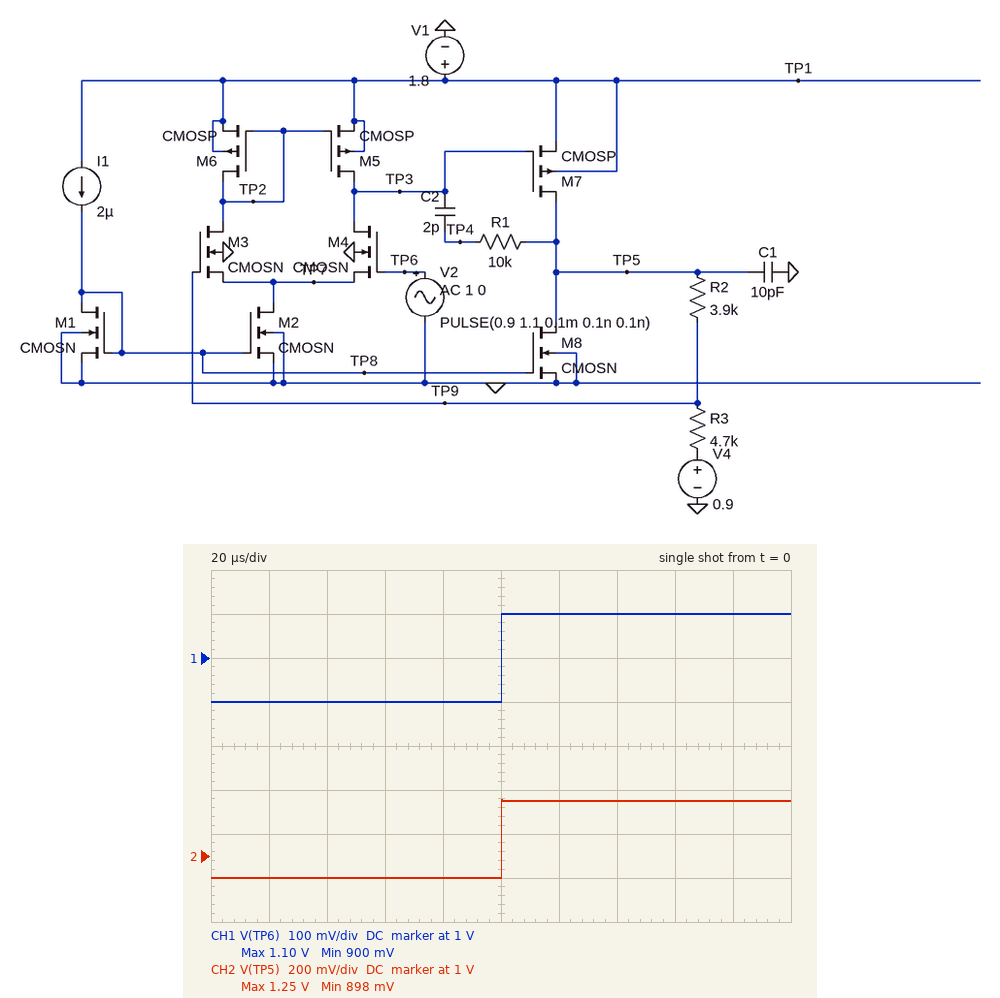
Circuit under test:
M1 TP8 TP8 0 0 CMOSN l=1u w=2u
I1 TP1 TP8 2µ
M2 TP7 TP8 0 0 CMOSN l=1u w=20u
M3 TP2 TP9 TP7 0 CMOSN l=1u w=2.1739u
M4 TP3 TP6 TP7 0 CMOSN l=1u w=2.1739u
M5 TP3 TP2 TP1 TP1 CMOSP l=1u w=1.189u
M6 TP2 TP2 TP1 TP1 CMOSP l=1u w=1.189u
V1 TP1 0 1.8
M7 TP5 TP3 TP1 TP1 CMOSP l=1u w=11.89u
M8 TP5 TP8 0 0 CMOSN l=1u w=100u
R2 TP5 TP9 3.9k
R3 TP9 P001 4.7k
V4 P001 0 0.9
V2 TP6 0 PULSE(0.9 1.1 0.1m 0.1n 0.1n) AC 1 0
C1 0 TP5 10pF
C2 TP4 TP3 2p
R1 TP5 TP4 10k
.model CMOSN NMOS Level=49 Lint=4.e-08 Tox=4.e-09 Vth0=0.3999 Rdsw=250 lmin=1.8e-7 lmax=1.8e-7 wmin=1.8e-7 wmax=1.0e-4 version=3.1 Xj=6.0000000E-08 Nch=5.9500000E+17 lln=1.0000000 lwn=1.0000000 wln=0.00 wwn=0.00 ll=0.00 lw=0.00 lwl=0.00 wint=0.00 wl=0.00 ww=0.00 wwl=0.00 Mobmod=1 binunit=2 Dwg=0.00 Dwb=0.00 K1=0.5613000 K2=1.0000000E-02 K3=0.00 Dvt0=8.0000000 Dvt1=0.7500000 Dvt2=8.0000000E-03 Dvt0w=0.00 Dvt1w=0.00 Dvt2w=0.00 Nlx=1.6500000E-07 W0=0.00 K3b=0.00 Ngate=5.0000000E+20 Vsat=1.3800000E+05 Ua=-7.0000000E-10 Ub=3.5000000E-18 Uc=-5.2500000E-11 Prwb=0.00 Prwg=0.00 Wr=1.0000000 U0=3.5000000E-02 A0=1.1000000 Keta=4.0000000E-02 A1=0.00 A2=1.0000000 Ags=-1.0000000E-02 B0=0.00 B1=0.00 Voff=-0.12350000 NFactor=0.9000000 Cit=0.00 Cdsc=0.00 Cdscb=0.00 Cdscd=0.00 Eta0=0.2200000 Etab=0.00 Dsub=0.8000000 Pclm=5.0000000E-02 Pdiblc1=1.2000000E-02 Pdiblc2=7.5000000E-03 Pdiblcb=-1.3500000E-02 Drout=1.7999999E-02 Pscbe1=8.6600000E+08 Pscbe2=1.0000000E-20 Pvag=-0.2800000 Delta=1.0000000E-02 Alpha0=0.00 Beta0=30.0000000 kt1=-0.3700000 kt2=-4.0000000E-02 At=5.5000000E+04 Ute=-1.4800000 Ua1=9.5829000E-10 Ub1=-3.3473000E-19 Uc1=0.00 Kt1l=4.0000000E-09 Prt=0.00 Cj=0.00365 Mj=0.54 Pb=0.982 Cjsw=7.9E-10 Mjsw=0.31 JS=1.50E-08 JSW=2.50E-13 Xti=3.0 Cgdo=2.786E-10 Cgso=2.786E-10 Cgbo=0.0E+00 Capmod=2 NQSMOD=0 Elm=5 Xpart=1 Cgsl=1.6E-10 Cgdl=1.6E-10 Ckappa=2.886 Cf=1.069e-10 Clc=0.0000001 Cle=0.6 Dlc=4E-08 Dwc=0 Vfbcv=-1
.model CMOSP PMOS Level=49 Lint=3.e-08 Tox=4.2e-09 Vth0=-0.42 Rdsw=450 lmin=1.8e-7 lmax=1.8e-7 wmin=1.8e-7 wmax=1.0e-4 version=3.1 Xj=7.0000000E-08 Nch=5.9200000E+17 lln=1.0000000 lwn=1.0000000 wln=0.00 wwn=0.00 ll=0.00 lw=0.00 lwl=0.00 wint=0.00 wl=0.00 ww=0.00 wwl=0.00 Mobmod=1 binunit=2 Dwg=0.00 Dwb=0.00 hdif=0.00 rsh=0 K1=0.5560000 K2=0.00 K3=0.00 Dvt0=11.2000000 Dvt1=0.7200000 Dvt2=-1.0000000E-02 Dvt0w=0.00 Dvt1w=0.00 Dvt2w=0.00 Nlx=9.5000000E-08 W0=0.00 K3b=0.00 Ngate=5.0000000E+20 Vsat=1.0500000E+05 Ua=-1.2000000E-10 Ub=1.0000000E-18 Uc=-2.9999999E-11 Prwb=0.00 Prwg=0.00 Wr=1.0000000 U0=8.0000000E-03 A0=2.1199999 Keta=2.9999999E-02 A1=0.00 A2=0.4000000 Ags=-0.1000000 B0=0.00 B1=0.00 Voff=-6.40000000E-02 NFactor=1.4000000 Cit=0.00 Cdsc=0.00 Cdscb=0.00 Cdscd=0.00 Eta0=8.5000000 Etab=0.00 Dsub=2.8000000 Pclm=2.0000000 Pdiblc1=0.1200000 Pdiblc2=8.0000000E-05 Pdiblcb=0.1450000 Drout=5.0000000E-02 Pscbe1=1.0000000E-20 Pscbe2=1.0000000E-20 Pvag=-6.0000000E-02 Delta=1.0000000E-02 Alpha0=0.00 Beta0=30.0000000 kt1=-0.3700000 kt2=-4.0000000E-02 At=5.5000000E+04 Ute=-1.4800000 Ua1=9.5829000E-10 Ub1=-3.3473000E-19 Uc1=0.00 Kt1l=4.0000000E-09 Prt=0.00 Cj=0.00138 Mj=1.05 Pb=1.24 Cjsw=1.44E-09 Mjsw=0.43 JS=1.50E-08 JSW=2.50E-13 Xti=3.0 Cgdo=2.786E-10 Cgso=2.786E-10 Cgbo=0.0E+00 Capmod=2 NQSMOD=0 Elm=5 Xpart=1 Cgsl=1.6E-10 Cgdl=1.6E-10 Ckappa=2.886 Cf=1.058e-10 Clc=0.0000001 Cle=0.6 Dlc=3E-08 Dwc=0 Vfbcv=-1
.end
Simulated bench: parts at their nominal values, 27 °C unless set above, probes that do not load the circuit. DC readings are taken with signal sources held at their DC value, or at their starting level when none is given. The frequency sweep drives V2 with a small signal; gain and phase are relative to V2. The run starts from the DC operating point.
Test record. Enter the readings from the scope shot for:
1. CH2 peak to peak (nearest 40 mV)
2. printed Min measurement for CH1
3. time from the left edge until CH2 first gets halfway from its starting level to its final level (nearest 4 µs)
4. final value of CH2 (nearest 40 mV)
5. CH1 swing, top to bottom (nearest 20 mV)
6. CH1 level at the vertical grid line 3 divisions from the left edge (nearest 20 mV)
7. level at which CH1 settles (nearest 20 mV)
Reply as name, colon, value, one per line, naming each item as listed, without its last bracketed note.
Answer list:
CH2 peak to peak: 360 mV
printed Min measurement for CH1: 900 mV
time from the left edge until CH2 first gets halfway from its starting level to its final level: 100 µs
final value of CH2: 1.24 V
CH1 swing, top to bottom: 200 mV
CH1 level at the vertical grid line 3 divisions from the left edge: 900 mV
level at which CH1 settles: 1.10 V
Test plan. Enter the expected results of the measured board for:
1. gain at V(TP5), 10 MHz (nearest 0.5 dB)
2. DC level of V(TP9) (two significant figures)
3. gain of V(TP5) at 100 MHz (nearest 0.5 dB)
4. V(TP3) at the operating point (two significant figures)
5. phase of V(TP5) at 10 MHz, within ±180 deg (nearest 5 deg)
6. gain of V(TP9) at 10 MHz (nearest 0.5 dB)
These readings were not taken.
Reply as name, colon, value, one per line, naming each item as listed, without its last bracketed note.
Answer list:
gain at V(TP5), 10 MHz: -10.5 dB
DC level of V(TP9): 900 mV
gain of V(TP5) at 100 MHz: -34.5 dB
V(TP3) at the operating point: 720 mV
phase of V(TP5) at 10 MHz, within ±180 deg: -100 deg
gain of V(TP9) at 10 MHz: -15.5 dB
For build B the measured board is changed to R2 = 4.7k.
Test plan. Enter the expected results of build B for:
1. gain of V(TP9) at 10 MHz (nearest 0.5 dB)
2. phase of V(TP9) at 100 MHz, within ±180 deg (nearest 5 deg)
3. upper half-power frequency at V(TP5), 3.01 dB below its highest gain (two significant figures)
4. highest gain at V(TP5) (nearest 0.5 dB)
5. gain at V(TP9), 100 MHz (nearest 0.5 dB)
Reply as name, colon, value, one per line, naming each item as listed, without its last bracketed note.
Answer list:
gain of V(TP9) at 10 MHz: -16.5 dB
phase of V(TP9) at 100 MHz, within ±180 deg: 150 deg
upper half-power frequency at V(TP5), 3.01 dB below its highest gain: 2.7 MHz
highest gain at V(TP5): 6.0 dB
gain at V(TP9), 100 MHz: -44.0 dB
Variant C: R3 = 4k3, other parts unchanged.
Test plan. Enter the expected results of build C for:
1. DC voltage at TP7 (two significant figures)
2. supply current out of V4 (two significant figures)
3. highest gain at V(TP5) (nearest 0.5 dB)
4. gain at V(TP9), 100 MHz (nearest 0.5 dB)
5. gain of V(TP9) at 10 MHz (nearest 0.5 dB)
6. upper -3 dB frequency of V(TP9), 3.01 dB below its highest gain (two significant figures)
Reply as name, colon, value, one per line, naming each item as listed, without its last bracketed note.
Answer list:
DC voltage at TP7: 220 mV
supply current out of V4: 170 nA
highest gain at V(TP5): 5.5 dB
gain at V(TP9), 100 MHz: -44.5 dB
gain of V(TP9) at 10 MHz: -16.0 dB
upper -3 dB frequency of V(TP9), 3.01 dB below its highest gain: 2.7 MHz
